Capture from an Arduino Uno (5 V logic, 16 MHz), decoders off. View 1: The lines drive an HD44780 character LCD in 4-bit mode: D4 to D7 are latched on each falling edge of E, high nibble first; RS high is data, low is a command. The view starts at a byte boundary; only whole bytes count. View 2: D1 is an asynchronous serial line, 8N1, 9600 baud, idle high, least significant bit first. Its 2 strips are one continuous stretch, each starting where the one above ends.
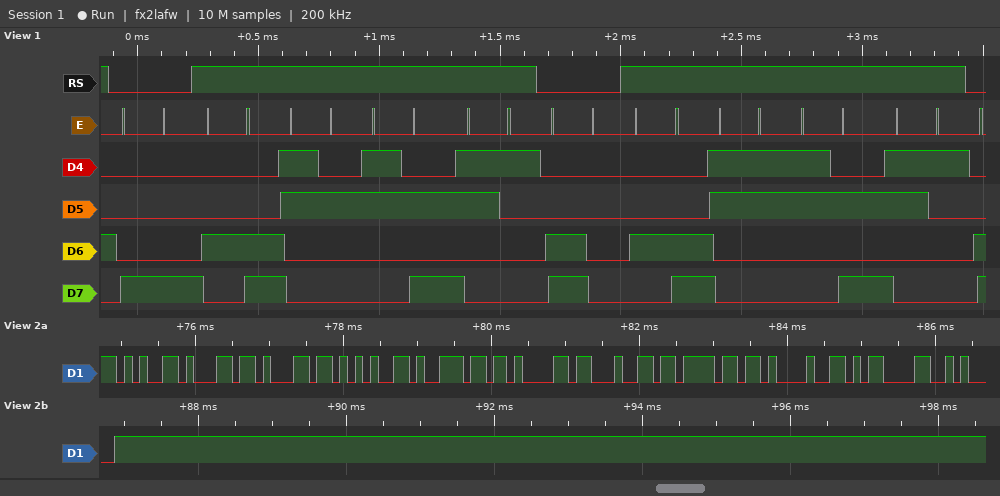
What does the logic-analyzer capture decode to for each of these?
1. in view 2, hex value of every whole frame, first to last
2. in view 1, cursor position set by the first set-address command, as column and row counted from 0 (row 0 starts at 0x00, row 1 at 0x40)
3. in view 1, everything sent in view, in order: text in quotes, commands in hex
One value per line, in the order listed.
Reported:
0x65 0x6C 0x6C 0x65 0x6E 0x61 0x64 0x6F 0x21 0x0D 0x0A
column 8, row 0
0x88 "L2:1" 0xC0 "L3:1"
